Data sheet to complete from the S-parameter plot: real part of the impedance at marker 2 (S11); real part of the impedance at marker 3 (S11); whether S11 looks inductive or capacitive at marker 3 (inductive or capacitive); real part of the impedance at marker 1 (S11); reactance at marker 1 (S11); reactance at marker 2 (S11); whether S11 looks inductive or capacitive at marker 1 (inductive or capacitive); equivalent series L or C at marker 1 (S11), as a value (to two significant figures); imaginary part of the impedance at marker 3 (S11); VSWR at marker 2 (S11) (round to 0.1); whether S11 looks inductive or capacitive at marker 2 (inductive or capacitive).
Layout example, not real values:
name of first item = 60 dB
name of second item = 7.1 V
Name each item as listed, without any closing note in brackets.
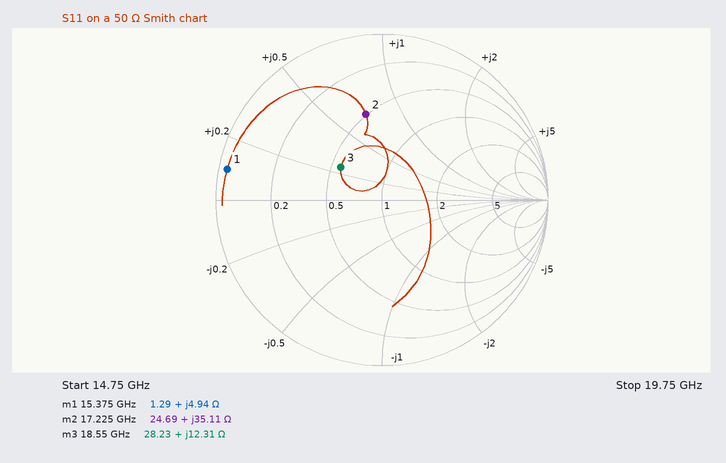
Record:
real part of the impedance at marker 2 = 24.69 Ω
real part of the impedance at marker 3 = 28.23 Ω
whether S11 looks inductive or capacitive at marker 3 = inductive
real part of the impedance at marker 1 = 1.29 Ω
reactance at marker 1 = +4.94 Ω
reactance at marker 2 = +35.11 Ω
whether S11 looks inductive or capacitive at marker 1 = inductive
equivalent series L or C at marker 1 (S11), as a value = 51 pH
imaginary part of the impedance at marker 3 = +12.31 Ω
VSWR at marker 2 (S11) = 3.2
whether S11 looks inductive or capacitive at marker 2 = inductive
